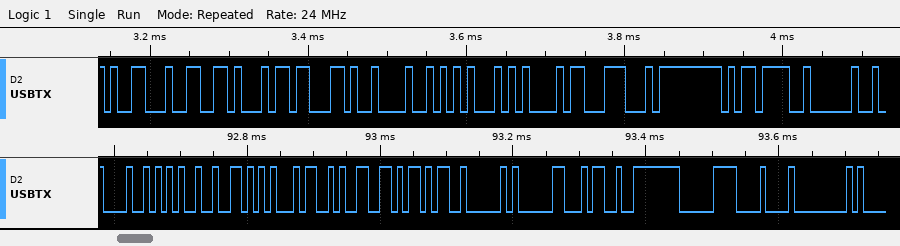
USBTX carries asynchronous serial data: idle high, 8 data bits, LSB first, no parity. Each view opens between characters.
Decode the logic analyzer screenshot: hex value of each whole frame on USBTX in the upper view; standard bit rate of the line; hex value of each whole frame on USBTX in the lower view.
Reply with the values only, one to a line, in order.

19, 66, B4, 2C, 48, 45, A1, 1C, FF, ED, 02
115200 baud
48, 25, 56, 34, 99, AD, 02, 81, 34, FE, E0, 08, 00
